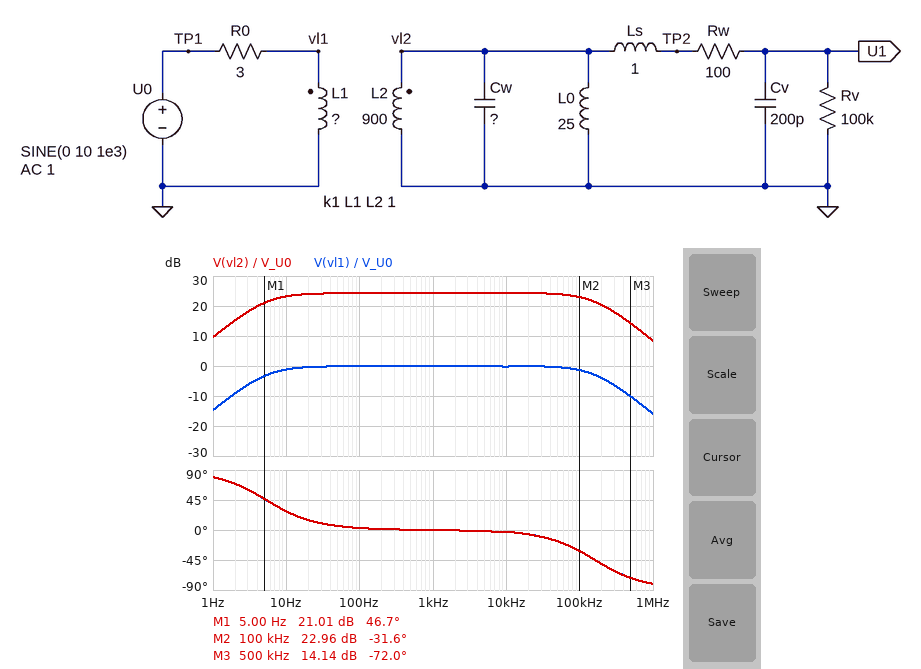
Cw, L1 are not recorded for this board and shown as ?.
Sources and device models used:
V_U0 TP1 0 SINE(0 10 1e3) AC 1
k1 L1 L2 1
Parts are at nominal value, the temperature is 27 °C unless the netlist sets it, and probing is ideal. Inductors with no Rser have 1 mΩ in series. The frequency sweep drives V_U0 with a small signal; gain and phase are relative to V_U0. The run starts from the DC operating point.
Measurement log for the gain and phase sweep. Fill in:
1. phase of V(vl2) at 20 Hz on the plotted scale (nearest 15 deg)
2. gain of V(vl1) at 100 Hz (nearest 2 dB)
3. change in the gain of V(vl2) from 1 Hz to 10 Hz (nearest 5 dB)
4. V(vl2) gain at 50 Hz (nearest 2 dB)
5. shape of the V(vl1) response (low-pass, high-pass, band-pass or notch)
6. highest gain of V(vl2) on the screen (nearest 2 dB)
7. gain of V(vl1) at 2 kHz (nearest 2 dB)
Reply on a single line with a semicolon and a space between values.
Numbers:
15 deg; 0 dB; 15 dB; 24 dB; band-pass; 24 dB; 0 dB
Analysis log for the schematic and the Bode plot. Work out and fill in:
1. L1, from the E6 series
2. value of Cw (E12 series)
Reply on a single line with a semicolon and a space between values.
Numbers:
3.3 H; 1.2 nF
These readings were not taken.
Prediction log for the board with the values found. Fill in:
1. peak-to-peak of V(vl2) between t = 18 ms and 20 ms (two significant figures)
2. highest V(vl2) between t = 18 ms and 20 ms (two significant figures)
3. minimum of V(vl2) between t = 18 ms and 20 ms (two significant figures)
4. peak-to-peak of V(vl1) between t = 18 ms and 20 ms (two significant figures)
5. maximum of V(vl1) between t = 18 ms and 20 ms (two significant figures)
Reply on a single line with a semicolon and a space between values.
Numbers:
330 V; 160 V; -160 V; 20 V; 9.9 V
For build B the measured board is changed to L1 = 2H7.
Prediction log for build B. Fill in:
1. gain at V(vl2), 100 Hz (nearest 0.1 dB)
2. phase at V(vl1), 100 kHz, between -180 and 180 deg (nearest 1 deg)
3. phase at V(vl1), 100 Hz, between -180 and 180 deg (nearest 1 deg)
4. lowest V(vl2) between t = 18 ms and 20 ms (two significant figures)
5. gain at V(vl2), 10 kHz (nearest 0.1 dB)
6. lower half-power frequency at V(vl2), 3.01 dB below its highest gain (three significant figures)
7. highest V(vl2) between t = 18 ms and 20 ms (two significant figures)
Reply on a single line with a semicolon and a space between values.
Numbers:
25.1 dB; -37 deg; 4 deg; -180 V; 25.0 dB; 6.48 Hz; 180 V
